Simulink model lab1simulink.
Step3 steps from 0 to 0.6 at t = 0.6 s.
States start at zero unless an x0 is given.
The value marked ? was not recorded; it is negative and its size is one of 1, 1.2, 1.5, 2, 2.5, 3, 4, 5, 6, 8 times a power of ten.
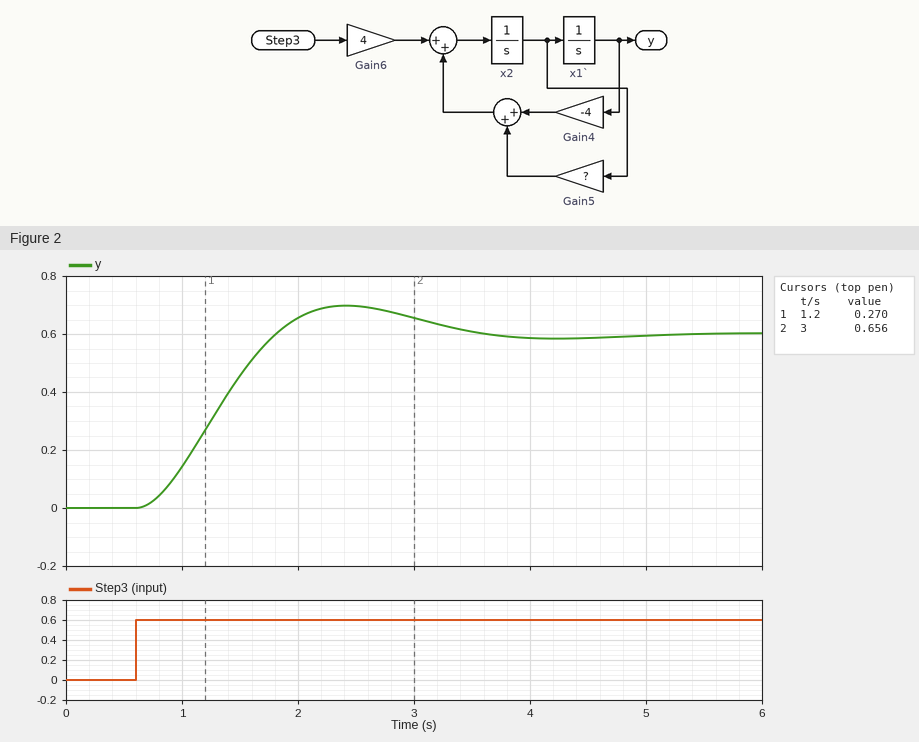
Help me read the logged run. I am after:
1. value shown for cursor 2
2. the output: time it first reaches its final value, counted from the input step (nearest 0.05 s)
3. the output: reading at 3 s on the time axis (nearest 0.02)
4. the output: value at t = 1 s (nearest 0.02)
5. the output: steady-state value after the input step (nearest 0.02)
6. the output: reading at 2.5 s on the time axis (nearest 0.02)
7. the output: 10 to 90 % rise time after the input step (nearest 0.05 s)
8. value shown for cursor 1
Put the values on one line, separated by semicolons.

0.656; 1.20 s; 0.66; 0.14; 0.60; 0.70; 0.80 s; 0.270
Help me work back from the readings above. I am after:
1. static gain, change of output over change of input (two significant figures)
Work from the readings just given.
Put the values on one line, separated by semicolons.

1.0
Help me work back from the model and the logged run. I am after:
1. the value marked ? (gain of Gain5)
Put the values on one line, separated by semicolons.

-2
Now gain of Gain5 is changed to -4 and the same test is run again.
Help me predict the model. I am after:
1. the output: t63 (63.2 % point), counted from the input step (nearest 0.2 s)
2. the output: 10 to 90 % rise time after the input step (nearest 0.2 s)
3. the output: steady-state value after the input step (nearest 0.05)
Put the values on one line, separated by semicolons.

1.0 s; 1.6 s; 0.60
